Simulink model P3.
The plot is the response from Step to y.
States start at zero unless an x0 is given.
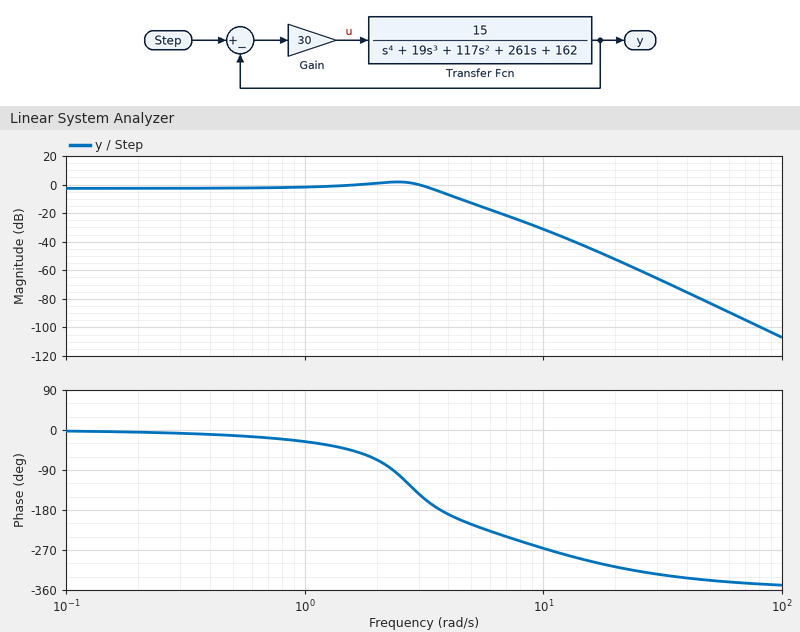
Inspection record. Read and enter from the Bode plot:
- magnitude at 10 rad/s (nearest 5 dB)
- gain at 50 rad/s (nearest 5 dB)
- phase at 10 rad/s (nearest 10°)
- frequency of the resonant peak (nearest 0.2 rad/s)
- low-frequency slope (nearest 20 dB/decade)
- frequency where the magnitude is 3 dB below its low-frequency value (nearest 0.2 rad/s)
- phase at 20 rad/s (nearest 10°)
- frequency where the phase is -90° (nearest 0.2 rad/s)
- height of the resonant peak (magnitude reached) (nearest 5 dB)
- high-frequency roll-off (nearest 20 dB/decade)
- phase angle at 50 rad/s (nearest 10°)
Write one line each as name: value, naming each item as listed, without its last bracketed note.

magnitude at 10 rad/s: -30 dB
gain at 50 rad/s: -85 dB
phase at 10 rad/s: -270°
frequency of the resonant peak: 2.4 rad/s
low-frequency slope: 0 dB/decade
frequency where the magnitude is 3 dB below its low-frequency value: 3.8 rad/s
phase at 20 rad/s: -310°
frequency where the phase is -90°: 2.4 rad/s
height of the resonant peak (magnitude reached): 0 dB
high-frequency roll-off: -80 dB/decade
phase angle at 50 rad/s: -340°
